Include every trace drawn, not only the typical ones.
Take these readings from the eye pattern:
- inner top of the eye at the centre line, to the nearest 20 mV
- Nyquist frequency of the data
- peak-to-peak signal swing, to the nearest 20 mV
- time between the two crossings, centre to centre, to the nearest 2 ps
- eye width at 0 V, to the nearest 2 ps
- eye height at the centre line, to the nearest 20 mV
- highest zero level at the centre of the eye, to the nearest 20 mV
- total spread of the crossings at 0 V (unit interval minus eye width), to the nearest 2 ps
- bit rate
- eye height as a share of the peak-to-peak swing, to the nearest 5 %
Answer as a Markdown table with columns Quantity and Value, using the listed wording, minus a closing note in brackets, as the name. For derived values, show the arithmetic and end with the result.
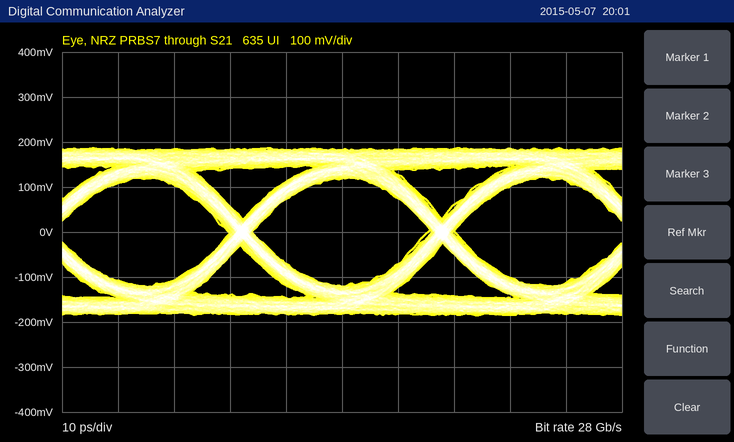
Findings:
| Quantity | Value |
|---|---|
| inner top of the eye at the centre line, to the nearest 20 mV | 120 mV |
| Nyquist frequency of the data | 14 GHz |
| peak-to-peak signal swing, to the nearest 20 mV | 380 mV |
| time between the two crossings, centre to centre, to the nearest 2 ps | 36 ps |
| eye width at 0 V, to the nearest 2 ps | 32 ps |
| eye height at the centre line, to the nearest 20 mV | 240 mV |
| highest zero level at the centre of the eye, to the nearest 20 mV | -120 mV |
| total spread of the crossings at 0 V (unit interval minus eye width), to the nearest 2 ps | 4 ps |
| bit rate | 28 Gb/s |
| eye height as a share of the peak-to-peak swing, to the nearest 5 % | 240 mV / 380 mV ≈ 63.2 %, so 65 % to the nearest 5 % |
